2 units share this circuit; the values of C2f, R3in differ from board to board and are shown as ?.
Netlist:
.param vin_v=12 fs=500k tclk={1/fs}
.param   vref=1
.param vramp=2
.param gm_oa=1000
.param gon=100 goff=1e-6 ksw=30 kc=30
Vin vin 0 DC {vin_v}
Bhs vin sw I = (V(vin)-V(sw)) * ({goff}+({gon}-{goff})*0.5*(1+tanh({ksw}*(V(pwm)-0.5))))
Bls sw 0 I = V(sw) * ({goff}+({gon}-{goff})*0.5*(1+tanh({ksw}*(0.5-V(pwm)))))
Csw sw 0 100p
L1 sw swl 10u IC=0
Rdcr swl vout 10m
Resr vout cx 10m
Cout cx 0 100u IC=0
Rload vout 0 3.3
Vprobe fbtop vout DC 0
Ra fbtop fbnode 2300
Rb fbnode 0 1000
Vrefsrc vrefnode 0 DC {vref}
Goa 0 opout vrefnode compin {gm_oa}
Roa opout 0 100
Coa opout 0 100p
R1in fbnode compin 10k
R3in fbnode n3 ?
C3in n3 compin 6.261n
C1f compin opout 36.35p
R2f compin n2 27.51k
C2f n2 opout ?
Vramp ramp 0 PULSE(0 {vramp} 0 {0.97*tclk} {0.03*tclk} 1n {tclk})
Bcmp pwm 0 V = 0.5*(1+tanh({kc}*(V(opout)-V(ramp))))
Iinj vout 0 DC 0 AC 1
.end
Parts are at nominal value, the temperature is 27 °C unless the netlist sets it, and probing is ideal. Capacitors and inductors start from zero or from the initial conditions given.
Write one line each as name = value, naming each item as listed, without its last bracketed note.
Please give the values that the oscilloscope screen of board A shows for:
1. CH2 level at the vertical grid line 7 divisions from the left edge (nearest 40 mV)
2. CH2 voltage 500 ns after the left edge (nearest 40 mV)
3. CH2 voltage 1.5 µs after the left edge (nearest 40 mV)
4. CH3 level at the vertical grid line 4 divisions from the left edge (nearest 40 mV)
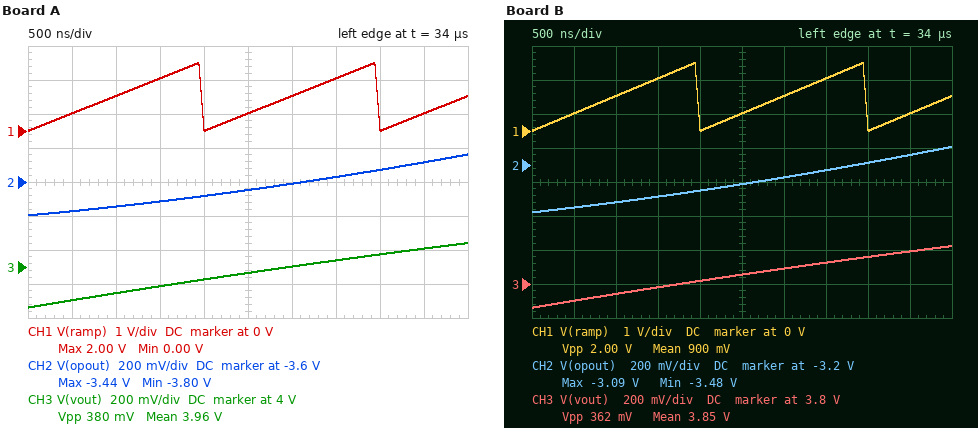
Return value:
CH2 level at the vertical grid line 7 divisions from the left edge = -3.56 V
CH2 voltage 500 ns after the left edge = -3.76 V
CH2 voltage 1.5 µs after the left edge = -3.72 V
CH3 level at the vertical grid line 4 divisions from the left edge = 3.92 V
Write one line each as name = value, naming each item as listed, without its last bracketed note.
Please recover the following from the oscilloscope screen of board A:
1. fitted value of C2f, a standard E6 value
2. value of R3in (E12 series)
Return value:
fitted value of C2f, a standard E6 value = 4.7 nF
value of R3in = 120 Ω
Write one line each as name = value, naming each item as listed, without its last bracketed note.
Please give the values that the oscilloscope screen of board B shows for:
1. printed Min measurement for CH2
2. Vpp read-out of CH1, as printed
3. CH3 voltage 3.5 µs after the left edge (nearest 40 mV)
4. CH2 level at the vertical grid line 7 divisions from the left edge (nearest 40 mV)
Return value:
printed Min measurement for CH2 = -3.48 V
Vpp read-out of CH1, as printed = 2.00 V
CH3 voltage 3.5 µs after the left edge = 3.92 V
CH2 level at the vertical grid line 7 divisions from the left edge = -3.24 V
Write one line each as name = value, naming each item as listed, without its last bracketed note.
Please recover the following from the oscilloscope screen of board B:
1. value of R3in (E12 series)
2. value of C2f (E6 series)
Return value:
value of R3in = 56 Ω
value of C2f = 4.7 nF
